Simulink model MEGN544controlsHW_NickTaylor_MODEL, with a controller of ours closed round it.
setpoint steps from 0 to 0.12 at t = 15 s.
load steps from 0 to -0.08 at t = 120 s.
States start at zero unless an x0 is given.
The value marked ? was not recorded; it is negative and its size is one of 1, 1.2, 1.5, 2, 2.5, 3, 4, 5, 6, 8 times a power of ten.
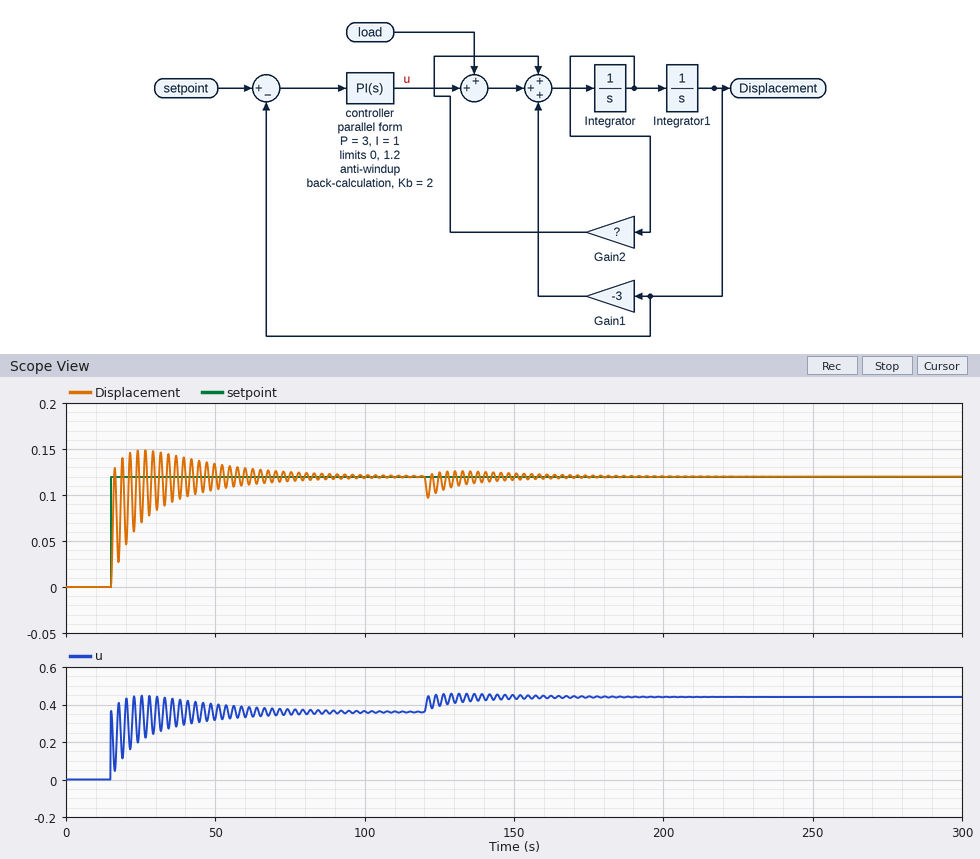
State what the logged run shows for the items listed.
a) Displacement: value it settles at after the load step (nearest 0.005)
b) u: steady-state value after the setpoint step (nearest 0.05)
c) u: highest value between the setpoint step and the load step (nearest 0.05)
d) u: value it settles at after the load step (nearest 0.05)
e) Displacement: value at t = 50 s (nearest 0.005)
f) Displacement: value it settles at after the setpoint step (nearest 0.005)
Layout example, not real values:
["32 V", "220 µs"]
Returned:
["0.120", "0.35", "0.45", "0.45", "0.130", "0.120"]
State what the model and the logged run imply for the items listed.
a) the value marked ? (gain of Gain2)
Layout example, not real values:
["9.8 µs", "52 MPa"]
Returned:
["-0.25"]
